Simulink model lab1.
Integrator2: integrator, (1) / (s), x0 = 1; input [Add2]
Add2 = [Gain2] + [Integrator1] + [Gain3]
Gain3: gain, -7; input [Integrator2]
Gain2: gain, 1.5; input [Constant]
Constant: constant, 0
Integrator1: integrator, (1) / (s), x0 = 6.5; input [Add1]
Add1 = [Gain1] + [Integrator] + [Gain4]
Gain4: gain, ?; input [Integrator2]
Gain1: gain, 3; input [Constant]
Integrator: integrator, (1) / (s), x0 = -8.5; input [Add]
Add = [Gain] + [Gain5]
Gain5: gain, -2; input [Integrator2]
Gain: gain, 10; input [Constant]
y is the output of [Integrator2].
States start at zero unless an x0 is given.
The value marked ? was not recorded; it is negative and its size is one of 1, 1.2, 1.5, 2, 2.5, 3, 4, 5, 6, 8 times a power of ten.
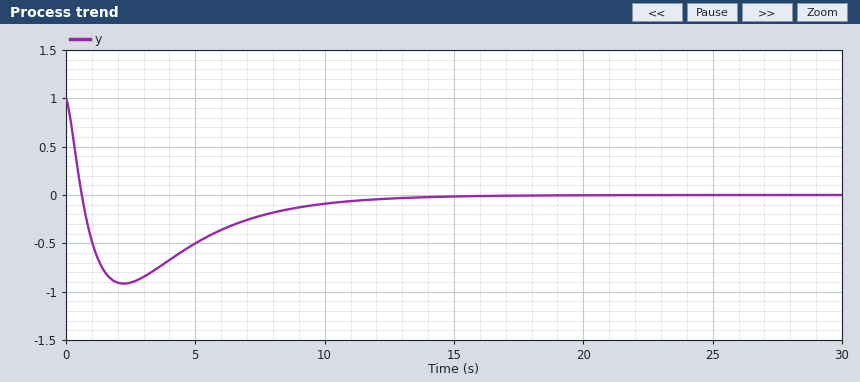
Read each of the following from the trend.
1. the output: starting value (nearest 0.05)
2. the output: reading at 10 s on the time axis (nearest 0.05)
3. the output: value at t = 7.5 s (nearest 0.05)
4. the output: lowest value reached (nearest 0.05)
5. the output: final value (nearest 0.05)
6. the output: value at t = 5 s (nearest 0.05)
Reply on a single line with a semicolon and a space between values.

1.00; -0.10; -0.20; -0.90; 0.00; -0.50
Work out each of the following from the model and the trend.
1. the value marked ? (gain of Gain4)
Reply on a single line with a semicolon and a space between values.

-8
